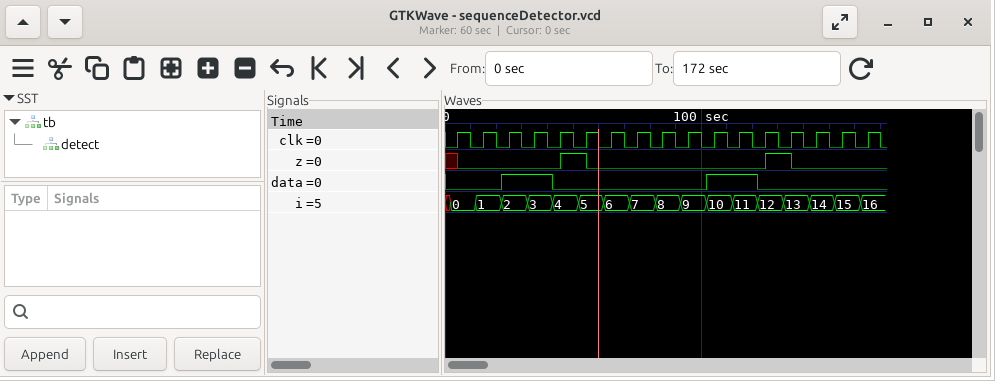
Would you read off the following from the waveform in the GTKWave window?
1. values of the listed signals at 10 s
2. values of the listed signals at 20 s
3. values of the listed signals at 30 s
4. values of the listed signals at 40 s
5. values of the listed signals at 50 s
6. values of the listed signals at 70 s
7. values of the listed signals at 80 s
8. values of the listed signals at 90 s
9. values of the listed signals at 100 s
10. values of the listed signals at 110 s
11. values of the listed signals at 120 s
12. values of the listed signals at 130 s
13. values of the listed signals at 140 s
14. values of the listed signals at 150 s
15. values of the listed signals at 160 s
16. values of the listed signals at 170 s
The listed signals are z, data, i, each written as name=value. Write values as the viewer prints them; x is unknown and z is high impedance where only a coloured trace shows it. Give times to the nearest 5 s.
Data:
z=0, data=0, i=0
z=0, data=0, i=1
z=0, data=1, i=2
z=0, data=1, i=3
z=1, data=0, i=4
z=0, data=0, i=6
z=0, data=0, i=7
z=0, data=0, i=8
z=0, data=0, i=9
z=0, data=1, i=10
z=0, data=1, i=11
z=1, data=0, i=12
z=0, data=0, i=13
z=0, data=0, i=14
z=0, data=0, i=15
z=0, data=0, i=16
